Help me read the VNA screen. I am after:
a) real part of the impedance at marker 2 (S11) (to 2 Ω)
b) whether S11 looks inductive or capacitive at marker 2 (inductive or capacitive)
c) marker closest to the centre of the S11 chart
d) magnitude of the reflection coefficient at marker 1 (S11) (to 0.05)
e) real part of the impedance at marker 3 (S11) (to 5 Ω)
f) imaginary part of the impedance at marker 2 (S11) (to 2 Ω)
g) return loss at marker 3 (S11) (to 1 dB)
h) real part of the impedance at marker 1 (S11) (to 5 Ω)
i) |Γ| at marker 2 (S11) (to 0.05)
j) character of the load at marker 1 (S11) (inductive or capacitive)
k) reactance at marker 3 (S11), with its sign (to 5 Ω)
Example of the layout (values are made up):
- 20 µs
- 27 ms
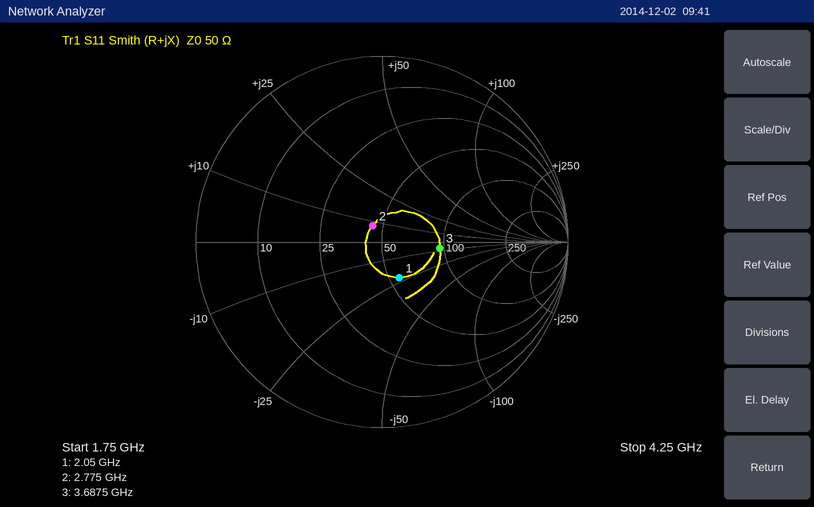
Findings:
- 44 Ω
- inductive
- marker 2
- 0.20
- 95 Ω
- +8 Ω
- 10 dB
- 55 Ω
- 0.10
- capacitive
- -5 Ω
